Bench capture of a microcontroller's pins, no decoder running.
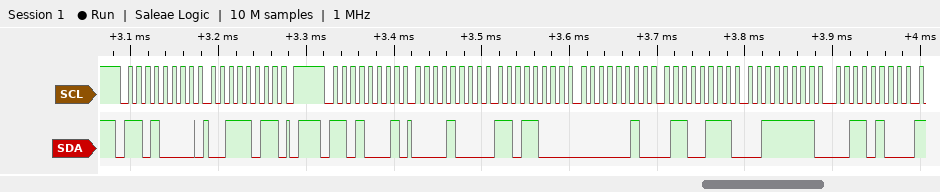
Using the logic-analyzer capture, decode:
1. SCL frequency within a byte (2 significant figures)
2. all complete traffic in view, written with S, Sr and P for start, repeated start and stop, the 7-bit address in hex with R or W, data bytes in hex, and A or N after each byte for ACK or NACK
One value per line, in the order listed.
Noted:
100 kHz
S 68W A 3B A P S 68R A 08 A D8 A 02 A 67 A 3F A 34 A
